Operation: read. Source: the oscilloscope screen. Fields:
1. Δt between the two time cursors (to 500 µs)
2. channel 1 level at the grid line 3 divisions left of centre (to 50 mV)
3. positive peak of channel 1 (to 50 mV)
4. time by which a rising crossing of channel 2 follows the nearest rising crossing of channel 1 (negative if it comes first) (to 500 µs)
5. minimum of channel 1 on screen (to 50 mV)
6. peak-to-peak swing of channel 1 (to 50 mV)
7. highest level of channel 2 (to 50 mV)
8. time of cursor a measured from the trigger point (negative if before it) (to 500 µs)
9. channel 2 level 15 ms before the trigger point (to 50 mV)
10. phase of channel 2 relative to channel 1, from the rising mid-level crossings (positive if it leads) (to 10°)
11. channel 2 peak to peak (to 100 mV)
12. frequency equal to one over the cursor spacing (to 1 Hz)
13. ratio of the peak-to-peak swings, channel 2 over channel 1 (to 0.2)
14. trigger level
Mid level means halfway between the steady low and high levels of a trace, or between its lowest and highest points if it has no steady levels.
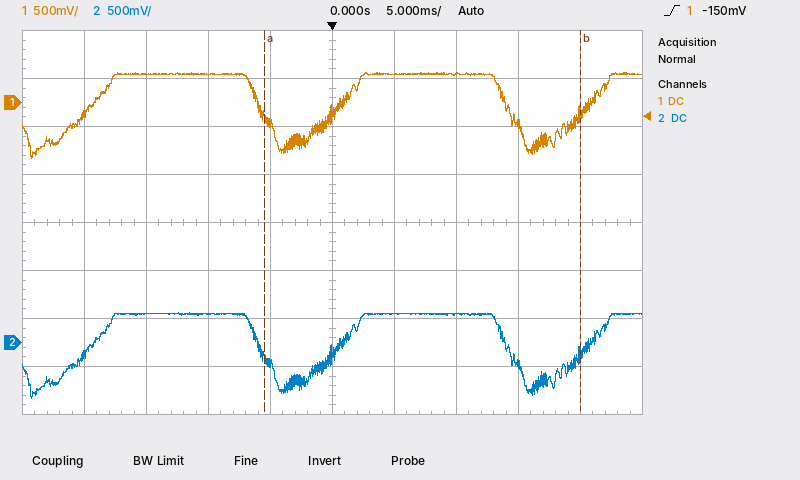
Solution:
25.5 ms
300 mV
300 mV
0.0 ms
-600 mV
900 mV
300 mV
-5.5 ms
300 mV
0°
900 mV
39 Hz
1.0
-150 mV
